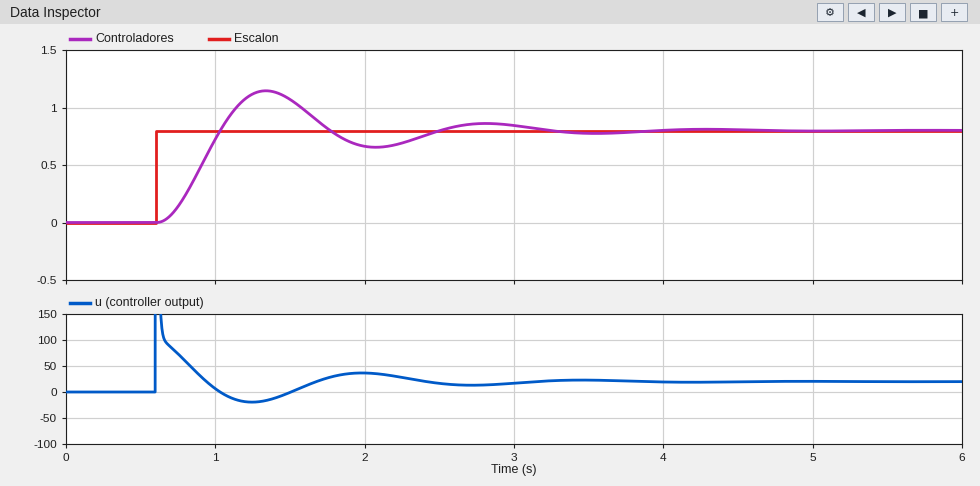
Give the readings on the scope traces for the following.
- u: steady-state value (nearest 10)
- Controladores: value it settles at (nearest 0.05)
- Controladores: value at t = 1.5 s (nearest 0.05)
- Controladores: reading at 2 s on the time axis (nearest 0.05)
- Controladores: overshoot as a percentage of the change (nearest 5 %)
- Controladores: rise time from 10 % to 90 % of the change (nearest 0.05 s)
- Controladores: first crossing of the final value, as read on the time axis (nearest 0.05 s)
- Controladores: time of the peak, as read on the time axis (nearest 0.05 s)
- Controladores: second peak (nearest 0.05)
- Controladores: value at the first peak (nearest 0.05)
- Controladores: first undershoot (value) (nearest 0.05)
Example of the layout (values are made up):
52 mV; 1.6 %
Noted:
20; 0.80; 1.05; 0.65; 45 %; 0.30 s; 1.05 s; 1.35 s; 0.85; 1.15; 0.65
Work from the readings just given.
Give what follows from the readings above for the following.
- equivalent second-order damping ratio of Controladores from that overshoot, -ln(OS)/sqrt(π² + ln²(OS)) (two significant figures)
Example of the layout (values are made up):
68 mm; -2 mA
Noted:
0.25
